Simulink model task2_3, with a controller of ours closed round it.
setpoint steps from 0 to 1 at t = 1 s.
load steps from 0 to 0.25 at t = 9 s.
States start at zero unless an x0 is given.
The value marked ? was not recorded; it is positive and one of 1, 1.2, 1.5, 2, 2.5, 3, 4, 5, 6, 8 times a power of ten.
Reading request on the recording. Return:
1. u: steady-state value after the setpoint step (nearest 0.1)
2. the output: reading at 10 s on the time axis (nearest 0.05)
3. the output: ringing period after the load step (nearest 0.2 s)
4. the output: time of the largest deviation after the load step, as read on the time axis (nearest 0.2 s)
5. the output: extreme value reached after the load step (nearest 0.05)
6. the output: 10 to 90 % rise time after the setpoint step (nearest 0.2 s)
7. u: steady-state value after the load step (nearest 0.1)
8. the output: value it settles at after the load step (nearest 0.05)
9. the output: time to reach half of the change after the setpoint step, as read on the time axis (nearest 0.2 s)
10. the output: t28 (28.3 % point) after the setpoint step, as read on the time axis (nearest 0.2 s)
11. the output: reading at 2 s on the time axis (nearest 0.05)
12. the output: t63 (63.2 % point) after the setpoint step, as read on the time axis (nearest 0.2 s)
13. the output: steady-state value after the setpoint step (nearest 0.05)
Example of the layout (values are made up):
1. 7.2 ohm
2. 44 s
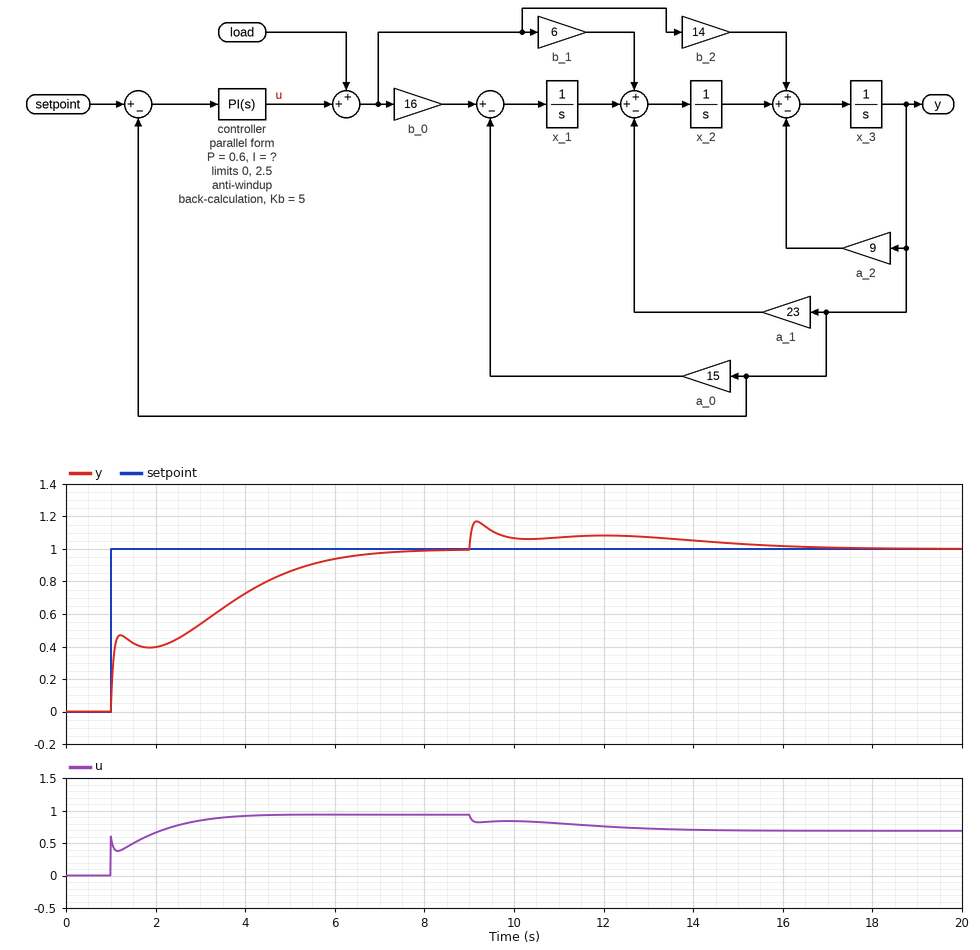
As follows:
1. 0.9
2. 1.05
3. 2.8 s
4. 9.2 s
5. 1.15
6. 4.4 s
7. 0.7
8. 1.00
9. 2.8 s
10. 1.0 s
11. 0.40
12. 3.4 s
13. 1.00
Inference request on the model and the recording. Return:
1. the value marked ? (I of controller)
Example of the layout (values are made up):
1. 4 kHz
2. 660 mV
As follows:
1. 0.5
